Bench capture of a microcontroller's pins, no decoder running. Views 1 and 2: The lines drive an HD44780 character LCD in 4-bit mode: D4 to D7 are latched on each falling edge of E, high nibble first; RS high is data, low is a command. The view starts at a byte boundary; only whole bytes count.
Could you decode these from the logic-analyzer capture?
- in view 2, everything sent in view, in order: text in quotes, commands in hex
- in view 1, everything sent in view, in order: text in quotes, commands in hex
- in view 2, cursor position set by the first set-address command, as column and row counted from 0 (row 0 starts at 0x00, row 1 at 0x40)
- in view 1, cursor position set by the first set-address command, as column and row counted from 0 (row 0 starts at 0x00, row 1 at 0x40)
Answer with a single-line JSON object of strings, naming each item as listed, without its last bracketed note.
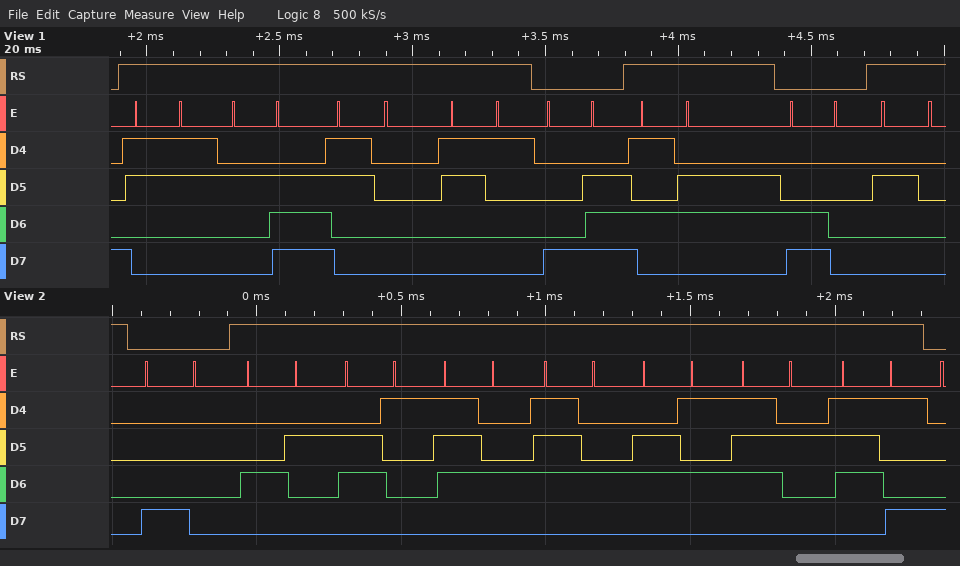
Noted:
{"in view 2, everything sent in view, in order: text in quotes, commands in hex": "0x80 \"Battery\"", "in view 1, everything sent in view, in order: text in quotes, commands in hex": "\"3.01\" 0x8E \"V\" 0xC0 \" \"", "in view 2, cursor position set by the first set-address command, as column and row counted from 0": "column 0, row 0", "in view 1, cursor position set by the first set-address command, as column and row counted from 0": "column 14, row 0"}
